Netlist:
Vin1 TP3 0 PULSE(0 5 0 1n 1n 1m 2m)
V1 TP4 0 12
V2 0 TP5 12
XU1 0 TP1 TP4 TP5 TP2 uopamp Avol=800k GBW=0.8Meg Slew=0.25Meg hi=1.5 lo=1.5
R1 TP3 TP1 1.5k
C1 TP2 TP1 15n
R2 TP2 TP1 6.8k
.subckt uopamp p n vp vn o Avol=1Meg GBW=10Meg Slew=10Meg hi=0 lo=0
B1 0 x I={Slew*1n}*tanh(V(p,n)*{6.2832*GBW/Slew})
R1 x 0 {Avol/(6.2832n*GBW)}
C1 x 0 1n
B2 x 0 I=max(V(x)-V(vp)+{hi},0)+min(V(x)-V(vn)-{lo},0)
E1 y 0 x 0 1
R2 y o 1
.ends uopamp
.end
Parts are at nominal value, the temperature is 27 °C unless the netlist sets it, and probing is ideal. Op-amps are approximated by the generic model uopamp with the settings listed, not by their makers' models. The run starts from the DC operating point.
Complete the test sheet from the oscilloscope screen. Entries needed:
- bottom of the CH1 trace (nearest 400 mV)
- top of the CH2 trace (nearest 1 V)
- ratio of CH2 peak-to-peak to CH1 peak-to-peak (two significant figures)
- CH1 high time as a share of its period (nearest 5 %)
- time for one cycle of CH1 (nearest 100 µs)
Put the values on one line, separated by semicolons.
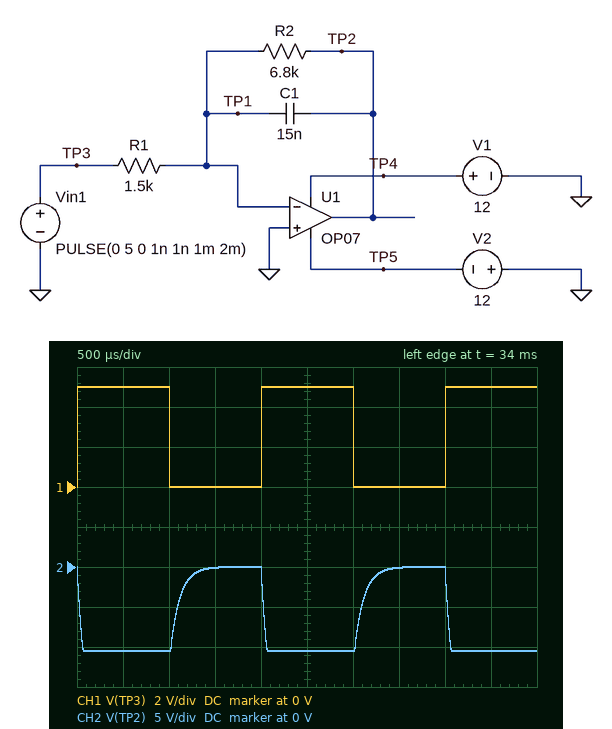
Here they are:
0 V; 0 V; 2.1; 50 %; 2.0 ms
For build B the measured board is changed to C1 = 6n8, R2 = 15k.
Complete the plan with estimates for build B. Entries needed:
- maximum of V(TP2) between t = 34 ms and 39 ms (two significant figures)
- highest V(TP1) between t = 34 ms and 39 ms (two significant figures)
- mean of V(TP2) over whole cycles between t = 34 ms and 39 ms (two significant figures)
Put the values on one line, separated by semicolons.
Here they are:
2.5 mV; 3.6 V; -5.8 V
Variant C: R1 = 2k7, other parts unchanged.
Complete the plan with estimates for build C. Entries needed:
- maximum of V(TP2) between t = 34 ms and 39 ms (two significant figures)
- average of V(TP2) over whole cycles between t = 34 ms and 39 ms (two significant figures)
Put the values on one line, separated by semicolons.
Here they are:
1.2 mV; -5.5 V
